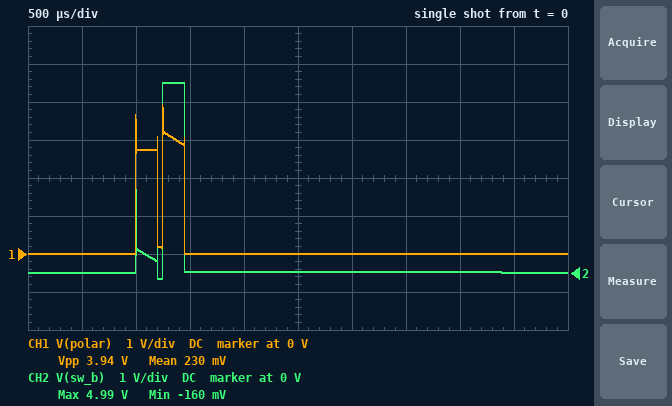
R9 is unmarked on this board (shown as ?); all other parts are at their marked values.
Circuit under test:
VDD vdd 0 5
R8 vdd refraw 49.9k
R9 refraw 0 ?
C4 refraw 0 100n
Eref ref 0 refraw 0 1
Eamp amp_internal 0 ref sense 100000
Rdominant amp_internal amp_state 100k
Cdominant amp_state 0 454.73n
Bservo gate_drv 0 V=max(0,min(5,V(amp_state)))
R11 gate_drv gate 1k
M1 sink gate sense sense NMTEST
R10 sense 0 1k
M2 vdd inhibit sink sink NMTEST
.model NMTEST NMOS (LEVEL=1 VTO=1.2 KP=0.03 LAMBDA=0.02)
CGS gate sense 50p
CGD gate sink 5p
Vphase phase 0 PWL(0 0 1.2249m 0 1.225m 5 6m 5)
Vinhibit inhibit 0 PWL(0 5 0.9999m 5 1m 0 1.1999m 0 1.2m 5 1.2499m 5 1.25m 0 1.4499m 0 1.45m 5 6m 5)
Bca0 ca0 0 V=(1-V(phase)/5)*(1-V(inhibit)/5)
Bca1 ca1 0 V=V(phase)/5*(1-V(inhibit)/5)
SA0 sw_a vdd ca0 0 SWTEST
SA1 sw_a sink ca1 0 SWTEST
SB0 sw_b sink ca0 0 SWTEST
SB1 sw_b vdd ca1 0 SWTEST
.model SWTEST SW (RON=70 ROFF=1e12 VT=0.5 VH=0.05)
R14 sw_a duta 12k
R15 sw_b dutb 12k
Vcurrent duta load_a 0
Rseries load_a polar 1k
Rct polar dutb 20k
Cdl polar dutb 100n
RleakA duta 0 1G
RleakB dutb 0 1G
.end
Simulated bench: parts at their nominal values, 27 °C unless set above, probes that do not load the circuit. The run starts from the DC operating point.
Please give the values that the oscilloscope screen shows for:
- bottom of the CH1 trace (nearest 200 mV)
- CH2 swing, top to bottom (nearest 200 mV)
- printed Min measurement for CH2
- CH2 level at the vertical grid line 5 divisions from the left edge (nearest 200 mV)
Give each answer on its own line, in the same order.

0 V
5.2 V
-160 mV
0 V
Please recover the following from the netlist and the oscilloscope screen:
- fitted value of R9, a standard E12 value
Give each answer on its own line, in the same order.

1.8 kΩ
